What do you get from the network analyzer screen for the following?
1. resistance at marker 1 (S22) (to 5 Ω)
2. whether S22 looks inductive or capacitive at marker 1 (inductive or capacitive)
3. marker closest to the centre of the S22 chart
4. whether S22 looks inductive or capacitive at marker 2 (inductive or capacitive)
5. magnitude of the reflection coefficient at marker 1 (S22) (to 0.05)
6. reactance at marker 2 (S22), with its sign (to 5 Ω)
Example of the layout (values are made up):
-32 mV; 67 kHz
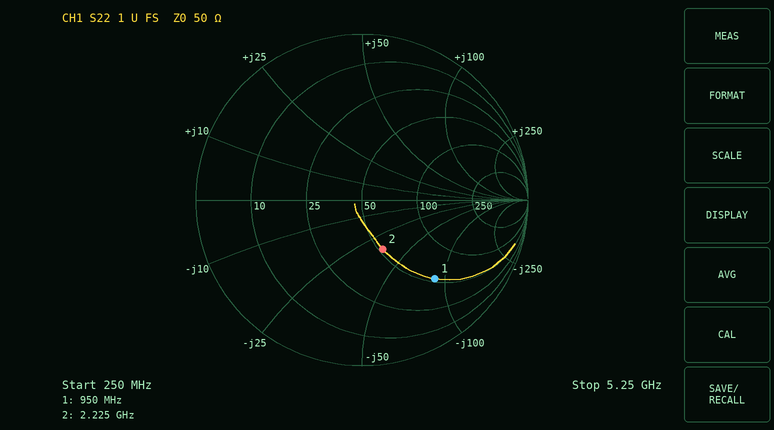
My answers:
55 Ω; capacitive; marker 2; capacitive; 0.65; -35 Ω
